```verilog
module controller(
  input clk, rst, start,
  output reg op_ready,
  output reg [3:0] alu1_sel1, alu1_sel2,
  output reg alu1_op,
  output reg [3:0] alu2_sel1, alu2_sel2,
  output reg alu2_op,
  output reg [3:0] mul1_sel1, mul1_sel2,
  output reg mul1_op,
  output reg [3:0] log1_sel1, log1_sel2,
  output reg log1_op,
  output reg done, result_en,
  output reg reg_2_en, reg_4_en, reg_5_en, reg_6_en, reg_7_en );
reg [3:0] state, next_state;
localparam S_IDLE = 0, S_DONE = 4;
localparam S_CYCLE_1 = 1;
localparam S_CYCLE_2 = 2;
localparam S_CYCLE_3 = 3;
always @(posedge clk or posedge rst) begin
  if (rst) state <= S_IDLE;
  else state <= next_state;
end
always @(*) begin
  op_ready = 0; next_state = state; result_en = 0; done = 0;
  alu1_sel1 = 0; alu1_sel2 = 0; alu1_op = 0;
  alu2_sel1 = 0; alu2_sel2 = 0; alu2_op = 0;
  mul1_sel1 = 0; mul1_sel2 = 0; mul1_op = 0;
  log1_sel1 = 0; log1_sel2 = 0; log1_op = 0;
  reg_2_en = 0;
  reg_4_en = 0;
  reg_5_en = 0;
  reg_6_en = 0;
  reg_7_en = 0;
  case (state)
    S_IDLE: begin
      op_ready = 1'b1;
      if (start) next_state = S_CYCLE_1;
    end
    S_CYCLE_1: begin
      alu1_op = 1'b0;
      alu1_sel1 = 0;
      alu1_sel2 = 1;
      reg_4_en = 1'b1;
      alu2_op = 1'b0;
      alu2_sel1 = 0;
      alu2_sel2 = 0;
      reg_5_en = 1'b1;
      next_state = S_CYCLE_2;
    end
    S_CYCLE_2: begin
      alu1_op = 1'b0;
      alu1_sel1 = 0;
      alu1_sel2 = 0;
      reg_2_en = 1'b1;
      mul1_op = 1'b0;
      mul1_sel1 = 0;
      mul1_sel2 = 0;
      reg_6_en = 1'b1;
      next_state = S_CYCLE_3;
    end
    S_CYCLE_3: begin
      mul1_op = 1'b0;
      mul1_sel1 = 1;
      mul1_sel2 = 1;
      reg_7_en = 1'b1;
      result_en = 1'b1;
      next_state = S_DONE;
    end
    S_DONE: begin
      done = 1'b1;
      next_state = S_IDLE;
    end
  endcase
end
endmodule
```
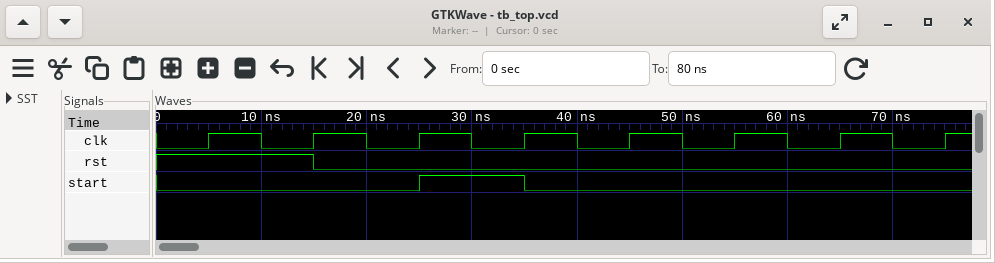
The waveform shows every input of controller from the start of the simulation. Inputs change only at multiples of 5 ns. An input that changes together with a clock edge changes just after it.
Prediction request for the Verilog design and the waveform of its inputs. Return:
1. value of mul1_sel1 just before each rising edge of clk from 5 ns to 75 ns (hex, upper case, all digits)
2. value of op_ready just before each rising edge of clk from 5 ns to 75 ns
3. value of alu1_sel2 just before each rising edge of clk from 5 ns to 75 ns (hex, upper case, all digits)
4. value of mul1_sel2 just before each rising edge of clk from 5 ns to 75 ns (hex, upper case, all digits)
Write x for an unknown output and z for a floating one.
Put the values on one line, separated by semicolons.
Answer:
0, 0, 0, 0, 0, 0, 1, 0; 1 1 1 1 0 0 0 0; 0, 0, 0, 0, 1, 0, 0, 0; 0, 0, 0, 0, 0, 0, 1, 0
